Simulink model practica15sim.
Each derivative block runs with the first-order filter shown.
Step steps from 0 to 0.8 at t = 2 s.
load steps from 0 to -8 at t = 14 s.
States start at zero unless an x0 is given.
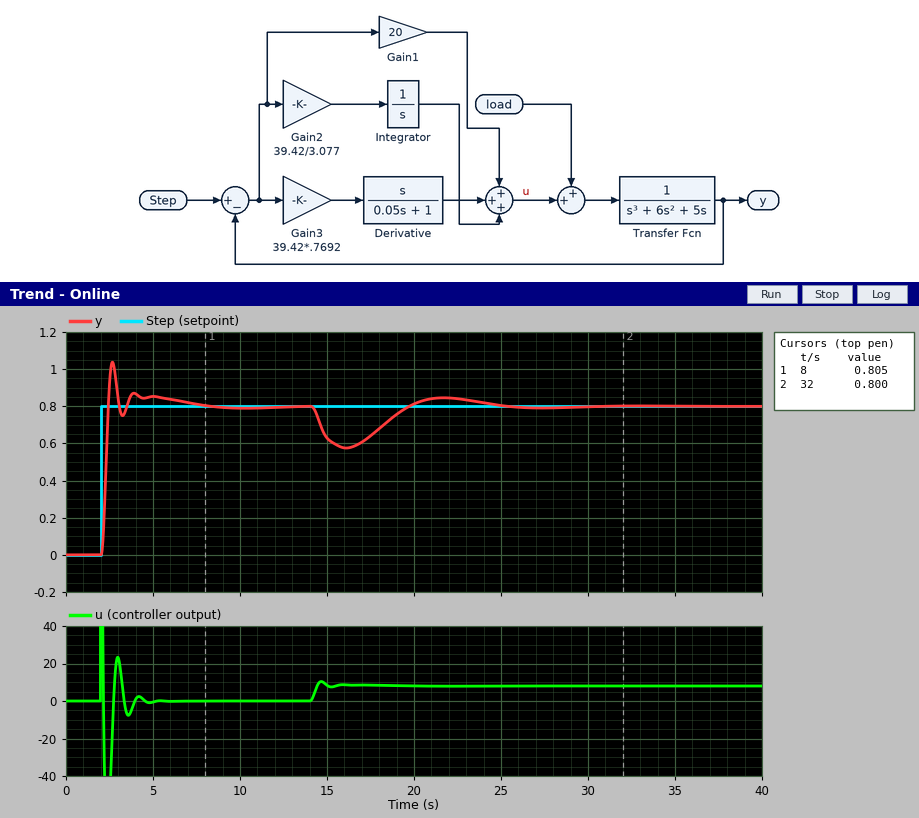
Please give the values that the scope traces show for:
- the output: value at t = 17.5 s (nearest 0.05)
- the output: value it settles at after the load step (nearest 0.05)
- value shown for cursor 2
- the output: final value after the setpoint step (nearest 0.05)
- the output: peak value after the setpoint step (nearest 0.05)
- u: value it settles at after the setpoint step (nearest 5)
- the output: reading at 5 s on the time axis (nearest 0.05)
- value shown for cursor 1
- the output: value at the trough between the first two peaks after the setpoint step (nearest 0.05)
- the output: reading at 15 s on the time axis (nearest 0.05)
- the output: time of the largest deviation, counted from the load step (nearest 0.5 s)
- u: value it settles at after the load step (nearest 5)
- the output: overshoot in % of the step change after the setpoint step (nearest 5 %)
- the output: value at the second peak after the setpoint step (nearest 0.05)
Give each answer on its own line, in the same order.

0.65
0.80
0.800
0.80
1.05
0
0.85
0.805
0.75
0.65
2.0 s
10
30 %
0.85
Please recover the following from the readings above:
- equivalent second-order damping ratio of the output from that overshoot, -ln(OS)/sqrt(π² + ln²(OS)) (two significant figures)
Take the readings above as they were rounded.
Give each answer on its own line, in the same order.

0.36
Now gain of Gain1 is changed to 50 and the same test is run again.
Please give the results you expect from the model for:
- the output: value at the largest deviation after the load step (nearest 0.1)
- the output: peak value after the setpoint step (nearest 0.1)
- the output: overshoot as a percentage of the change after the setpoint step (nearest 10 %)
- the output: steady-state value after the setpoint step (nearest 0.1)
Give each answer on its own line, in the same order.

0.7
1.2
50 %
0.8
